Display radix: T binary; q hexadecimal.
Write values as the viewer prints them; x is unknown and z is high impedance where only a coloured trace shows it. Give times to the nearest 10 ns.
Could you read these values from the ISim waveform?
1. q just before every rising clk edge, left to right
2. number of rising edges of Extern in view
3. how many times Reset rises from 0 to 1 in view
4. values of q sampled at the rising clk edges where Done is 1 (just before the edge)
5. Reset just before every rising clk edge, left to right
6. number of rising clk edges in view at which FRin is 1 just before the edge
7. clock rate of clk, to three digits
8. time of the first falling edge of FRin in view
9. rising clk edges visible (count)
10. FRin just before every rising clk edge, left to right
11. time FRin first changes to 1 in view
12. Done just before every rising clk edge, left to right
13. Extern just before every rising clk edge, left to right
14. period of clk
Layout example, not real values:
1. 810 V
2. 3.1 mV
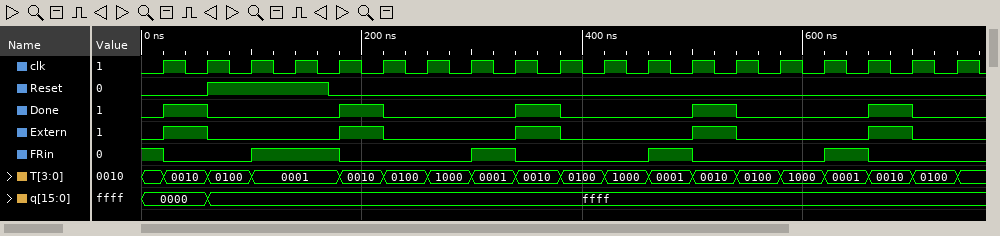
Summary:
1. 0000, 0000, ffff, ffff, ffff, ffff, ffff, ffff, ffff, ffff, ffff, ffff, ffff, ffff, ffff, ffff, ffff, ffff, ffff
2. 5
3. 1
4. 0000, ffff, ffff, ffff, ffff
5. 0 0 1 1 0 0 0 0 0 0 0 0 0 0 0 0 0 0 0
6. 6
7. 25.0 MHz
8. 20 ns
9. 19
10. 1 0 0 1 1 0 0 0 1 0 0 0 1 0 0 0 1 0 0
11. 100 ns
12. 0 1 0 0 0 1 0 0 0 1 0 0 0 1 0 0 0 1 0
13. 0 1 0 0 0 1 0 0 0 1 0 0 0 1 0 0 0 1 0
14. 40 ns
